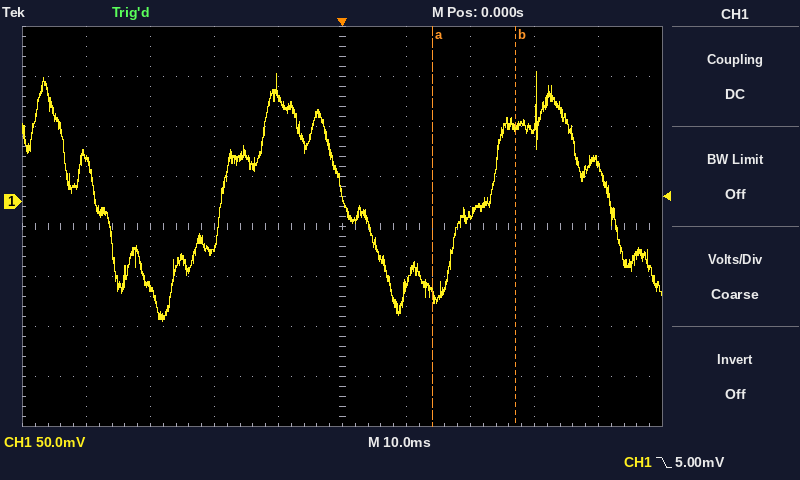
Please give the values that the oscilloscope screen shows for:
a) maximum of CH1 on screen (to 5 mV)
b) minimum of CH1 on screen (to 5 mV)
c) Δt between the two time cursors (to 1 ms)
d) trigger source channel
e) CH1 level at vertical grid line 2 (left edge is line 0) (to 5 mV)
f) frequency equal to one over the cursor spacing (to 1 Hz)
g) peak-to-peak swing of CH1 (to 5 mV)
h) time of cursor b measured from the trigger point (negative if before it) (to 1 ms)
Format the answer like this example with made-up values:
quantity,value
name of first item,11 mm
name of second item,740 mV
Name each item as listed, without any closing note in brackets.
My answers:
quantity,value
maximum of CH1 on screen,130 mV
minimum of CH1 on screen,-120 mV
Δt between the two time cursors,13 ms
trigger source channel,CH1
CH1 level at vertical grid line 2 (left edge is line 0),-85 mV
frequency equal to one over the cursor spacing,77 Hz
peak-to-peak swing of CH1,250 mV
time of cursor b measured from the trigger point (negative if before it),+27 ms
